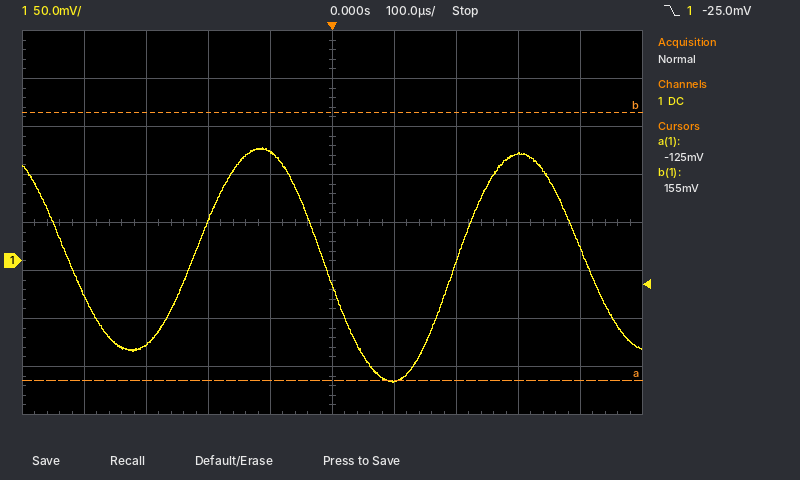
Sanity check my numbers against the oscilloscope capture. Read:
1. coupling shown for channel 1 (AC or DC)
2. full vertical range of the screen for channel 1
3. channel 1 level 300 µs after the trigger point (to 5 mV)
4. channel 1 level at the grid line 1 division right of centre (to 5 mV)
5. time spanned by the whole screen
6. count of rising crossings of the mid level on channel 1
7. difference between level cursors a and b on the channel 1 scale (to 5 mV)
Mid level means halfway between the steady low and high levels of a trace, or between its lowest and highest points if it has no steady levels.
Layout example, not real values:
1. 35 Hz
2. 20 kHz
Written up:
1. DC
2. 400 mV
3. 110 mV
4. -125 mV
5. 1 ms
6. 2
7. 280 mV
